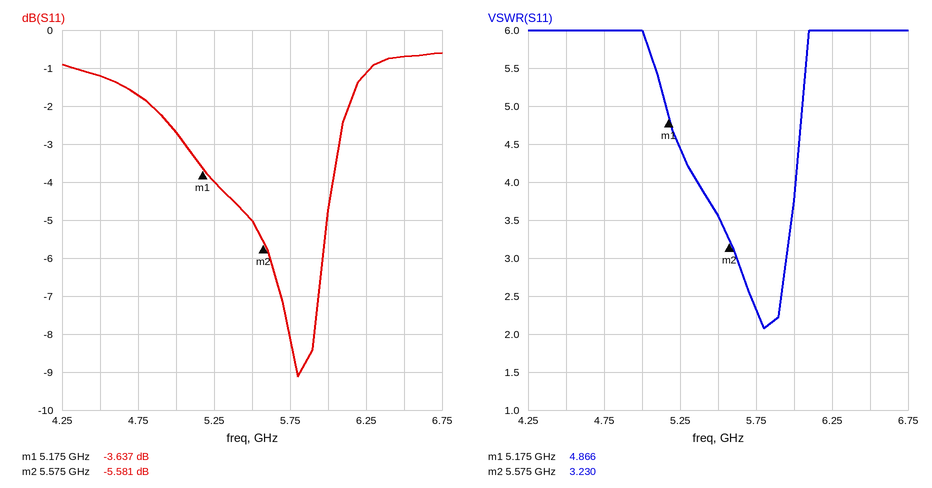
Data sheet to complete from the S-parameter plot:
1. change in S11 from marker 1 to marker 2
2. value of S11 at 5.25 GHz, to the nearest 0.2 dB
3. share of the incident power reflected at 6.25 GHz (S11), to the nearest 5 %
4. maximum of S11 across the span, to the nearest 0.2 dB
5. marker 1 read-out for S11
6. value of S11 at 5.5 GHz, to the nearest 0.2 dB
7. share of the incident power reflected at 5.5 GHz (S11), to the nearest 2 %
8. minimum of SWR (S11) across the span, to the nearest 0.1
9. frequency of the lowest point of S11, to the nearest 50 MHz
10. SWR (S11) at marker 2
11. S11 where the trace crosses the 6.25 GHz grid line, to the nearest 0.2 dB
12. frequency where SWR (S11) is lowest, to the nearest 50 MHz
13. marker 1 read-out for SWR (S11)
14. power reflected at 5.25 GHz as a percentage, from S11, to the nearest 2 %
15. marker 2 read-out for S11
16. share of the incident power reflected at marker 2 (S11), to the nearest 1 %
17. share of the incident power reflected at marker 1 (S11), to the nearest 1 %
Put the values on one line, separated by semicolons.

-1.944 dB; -4.0 dB; 75 %; -0.6 dB; -3.637 dB; -5.0 dB; 32 %; 2.1; 5.80 GHz; 3.230; -1.2 dB; 5.80 GHz; 4.866; 40 %; -5.581 dB; 28 %; 43 %
